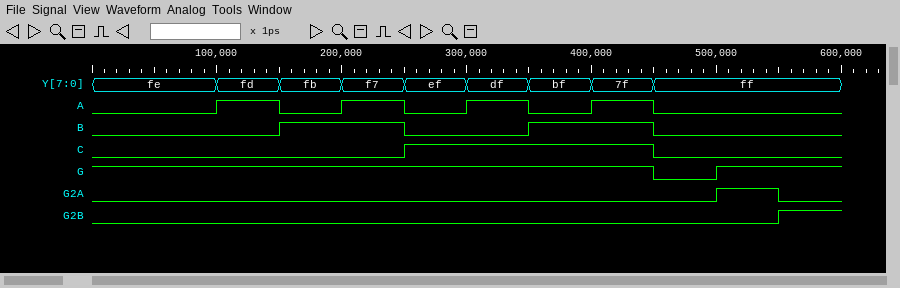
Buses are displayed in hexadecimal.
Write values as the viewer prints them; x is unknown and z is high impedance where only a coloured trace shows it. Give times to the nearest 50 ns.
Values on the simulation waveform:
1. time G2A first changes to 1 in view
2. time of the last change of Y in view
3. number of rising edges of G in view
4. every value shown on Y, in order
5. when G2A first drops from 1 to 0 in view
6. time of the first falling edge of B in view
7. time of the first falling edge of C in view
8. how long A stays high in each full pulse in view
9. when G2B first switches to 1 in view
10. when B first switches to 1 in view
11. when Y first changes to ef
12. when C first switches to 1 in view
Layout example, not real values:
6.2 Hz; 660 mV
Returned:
500 ns; 450 ns; 1; fe, fd, fb, f7, ef, df, bf, 7f, ff; 550 ns; 250 ns; 450 ns; 50 ns, 50 ns, 50 ns, 50 ns; 550 ns; 150 ns; 250 ns; 250 ns
